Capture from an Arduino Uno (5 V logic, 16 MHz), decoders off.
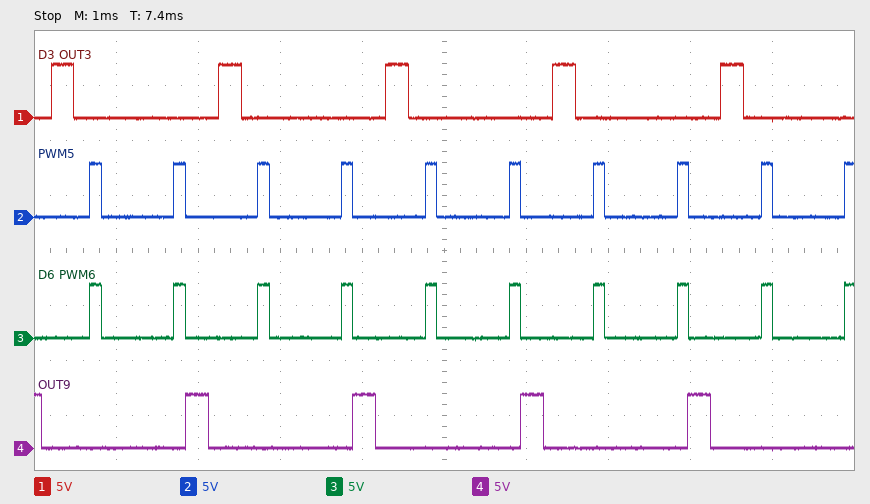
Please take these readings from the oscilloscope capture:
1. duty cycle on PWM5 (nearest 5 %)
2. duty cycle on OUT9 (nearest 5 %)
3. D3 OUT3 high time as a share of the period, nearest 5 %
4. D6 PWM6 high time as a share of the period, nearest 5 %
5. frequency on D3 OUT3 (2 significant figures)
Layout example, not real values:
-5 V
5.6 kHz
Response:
15 %
15 %
15 %
15 %
490 Hz
